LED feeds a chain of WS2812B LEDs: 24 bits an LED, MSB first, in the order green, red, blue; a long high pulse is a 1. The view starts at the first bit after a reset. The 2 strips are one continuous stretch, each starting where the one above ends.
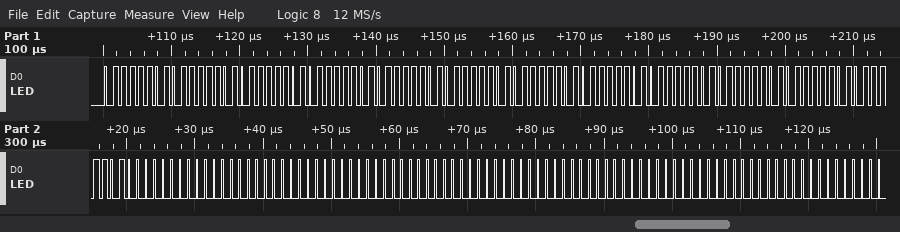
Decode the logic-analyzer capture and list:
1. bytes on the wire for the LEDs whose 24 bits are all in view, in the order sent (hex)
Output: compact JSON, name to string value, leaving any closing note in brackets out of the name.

{"bytes on the wire for the LEDs whose 24 bits are all in view, in the order sent": "7D 7D 7D 7D 7D 7D 7D 7D 7D 7D 7D 7D 00 00 00 00 00 00 00 00 00"}
